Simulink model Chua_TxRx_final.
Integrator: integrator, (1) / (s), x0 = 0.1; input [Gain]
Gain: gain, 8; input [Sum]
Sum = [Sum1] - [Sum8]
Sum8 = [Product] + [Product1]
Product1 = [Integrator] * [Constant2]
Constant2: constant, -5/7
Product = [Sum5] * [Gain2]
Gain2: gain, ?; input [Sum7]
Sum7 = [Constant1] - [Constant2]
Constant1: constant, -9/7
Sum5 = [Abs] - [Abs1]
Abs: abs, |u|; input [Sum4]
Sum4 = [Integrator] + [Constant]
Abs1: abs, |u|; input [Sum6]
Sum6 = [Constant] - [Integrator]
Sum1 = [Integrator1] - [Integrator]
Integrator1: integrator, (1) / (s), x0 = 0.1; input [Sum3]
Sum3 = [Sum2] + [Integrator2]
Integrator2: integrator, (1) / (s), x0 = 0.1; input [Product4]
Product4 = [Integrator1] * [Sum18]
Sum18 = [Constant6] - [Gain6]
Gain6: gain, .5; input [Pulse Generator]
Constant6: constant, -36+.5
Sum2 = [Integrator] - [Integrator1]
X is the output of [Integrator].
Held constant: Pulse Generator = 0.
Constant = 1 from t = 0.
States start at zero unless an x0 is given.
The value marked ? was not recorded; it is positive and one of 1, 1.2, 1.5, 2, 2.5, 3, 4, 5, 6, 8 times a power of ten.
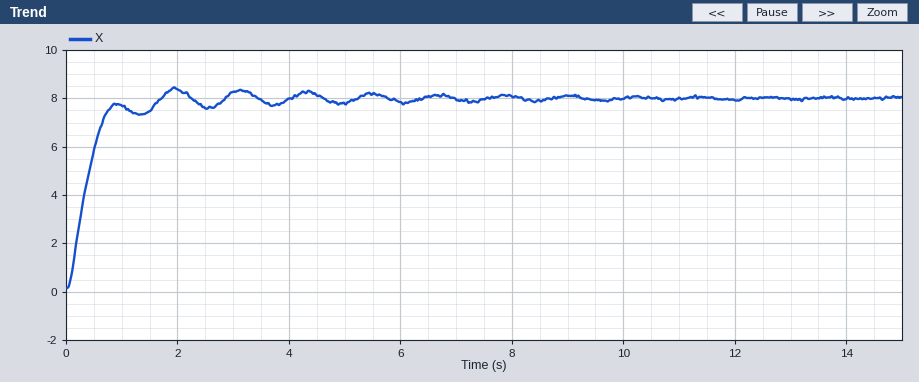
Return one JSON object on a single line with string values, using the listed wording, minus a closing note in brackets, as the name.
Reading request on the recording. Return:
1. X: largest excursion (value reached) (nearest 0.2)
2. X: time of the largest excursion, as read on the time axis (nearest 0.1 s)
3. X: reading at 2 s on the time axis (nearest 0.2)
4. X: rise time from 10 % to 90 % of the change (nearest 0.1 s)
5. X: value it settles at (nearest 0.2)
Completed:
{"X: largest excursion (value reached)": "8.4", "X: time of the largest excursion, as read on the time axis": "2.0 s", "X: reading at 2 s on the time axis": "8.4", "X: rise time from 10 % to 90 % of the change": "0.6 s", "X: value it settles at": "8.0"}
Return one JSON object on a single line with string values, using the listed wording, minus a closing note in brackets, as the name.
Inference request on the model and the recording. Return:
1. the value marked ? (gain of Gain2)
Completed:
{"the value marked ?": "2"}
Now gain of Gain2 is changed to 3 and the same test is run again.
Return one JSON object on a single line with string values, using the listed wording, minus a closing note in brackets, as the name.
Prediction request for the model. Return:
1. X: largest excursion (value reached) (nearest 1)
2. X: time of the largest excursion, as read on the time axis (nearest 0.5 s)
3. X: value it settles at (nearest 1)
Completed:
{"X: largest excursion (value reached)": "13", "X: time of the largest excursion, as read on the time axis": "2.0 s", "X: value it settles at": "12"}
